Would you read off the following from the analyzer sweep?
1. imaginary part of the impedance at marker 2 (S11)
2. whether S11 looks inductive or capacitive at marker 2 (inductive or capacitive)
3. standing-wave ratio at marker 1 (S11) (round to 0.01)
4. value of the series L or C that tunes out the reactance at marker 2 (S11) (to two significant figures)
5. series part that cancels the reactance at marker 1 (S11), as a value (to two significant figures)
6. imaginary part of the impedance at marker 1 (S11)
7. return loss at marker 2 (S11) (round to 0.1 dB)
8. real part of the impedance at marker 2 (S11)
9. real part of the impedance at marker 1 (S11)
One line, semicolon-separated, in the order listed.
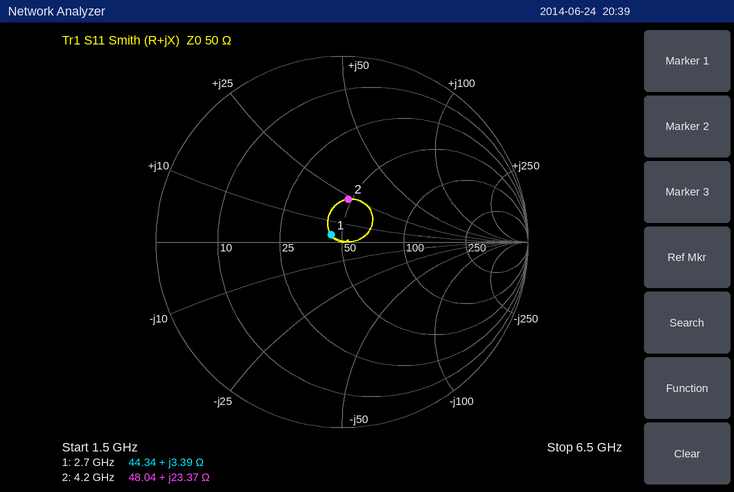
+23.37 Ω; inductive; 1.15; 1.6 pF; 17 pF; +3.39 Ω; 12.7 dB; 48.04 Ω; 44.34 Ω
